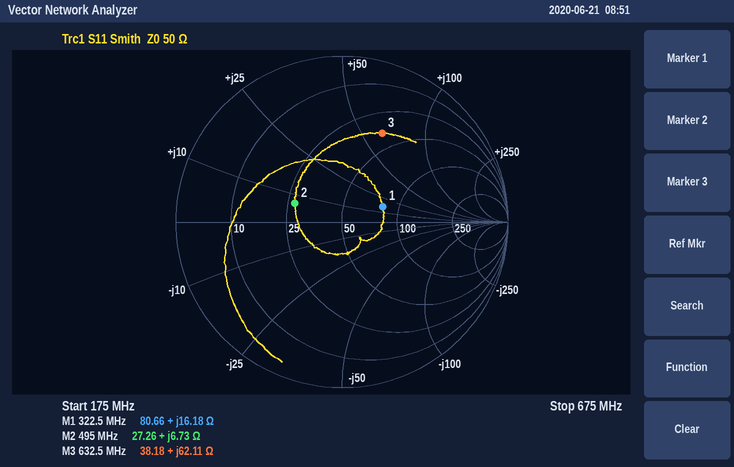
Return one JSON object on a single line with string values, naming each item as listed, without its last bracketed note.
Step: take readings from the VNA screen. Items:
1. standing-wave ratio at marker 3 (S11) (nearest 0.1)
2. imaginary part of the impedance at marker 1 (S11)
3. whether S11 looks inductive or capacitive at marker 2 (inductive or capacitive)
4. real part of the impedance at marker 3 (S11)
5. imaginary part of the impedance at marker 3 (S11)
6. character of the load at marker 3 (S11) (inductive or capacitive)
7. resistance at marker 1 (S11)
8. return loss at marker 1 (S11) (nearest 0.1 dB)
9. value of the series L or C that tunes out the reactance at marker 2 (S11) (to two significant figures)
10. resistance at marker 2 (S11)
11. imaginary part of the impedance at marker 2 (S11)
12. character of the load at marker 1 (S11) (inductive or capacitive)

{"standing-wave ratio at marker 3 (S11)": "3.8", "imaginary part of the impedance at marker 1": "+16.18 Ω", "whether S11 looks inductive or capacitive at marker 2": "inductive", "real part of the impedance at marker 3": "38.18 Ω", "imaginary part of the impedance at marker 3": "+62.11 Ω", "character of the load at marker 3 (S11)": "inductive", "resistance at marker 1": "80.66 Ω", "return loss at marker 1 (S11)": "11.6 dB", "value of the series L or C that tunes out the reactance at marker 2 (S11)": "48 pF", "resistance at marker 2": "27.26 Ω", "imaginary part of the impedance at marker 2": "+6.73 Ω", "character of the load at marker 1 (S11)": "inductive"}
